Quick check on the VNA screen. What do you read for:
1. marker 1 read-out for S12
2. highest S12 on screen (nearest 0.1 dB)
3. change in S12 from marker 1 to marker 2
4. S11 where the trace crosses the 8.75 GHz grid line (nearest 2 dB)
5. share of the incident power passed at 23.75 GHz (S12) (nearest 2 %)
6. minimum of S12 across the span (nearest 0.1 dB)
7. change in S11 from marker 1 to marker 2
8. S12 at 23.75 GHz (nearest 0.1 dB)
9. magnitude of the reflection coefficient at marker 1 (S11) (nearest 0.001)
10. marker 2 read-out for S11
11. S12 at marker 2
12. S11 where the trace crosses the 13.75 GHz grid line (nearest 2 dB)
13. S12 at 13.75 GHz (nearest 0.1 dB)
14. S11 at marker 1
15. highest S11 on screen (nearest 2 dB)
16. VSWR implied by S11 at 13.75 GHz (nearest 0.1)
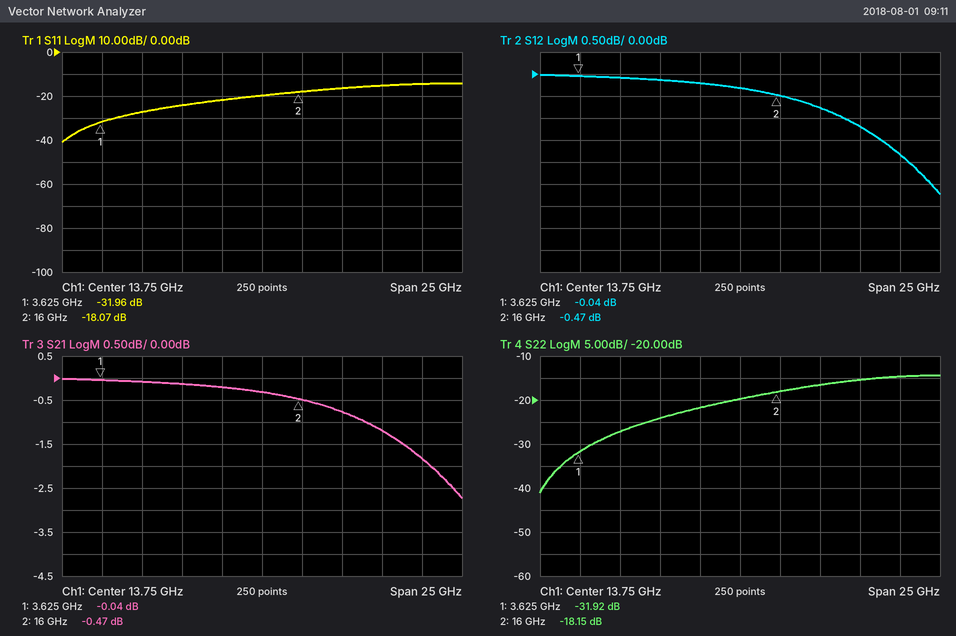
-0.04 dB
0.0 dB
-0.43 dB
-24 dB
66 %
-2.7 dB
13.89 dB
-1.8 dB
0.025
-18.07 dB
-0.47 dB
-20 dB
-0.3 dB
-31.96 dB
-14 dB
1.2
